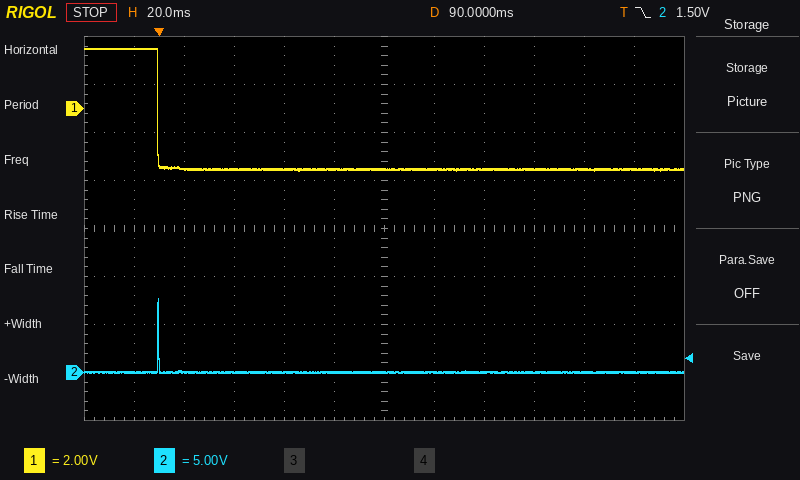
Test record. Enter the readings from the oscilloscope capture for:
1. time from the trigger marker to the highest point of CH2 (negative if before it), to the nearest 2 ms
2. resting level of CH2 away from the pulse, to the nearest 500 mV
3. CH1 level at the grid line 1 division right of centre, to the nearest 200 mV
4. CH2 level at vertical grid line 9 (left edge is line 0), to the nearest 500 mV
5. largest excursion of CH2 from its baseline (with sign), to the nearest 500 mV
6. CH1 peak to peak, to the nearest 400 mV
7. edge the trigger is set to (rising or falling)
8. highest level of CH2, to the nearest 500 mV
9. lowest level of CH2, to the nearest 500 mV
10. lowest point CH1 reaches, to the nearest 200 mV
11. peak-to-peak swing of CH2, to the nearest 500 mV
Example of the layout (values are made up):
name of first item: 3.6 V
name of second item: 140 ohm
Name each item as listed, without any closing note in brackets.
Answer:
time from the trigger marker to the highest point of CH2 (negative if before it), to the nearest 2 ms: 0 ms
resting level of CH2 away from the pulse, to the nearest 500 mV: 0.0 V
CH1 level at the grid line 1 division right of centre, to the nearest 200 mV: -2.6 V
CH2 level at vertical grid line 9 (left edge is line 0), to the nearest 500 mV: 0.0 V
largest excursion of CH2 from its baseline (with sign), to the nearest 500 mV: +7.5 V
CH1 peak to peak, to the nearest 400 mV: 5.2 V
edge the trigger is set to: falling
highest level of CH2, to the nearest 500 mV: 7.5 V
lowest level of CH2, to the nearest 500 mV: 0.0 V
lowest point CH1 reaches, to the nearest 200 mV: -2.6 V
peak-to-peak swing of CH2, to the nearest 500 mV: 7.5 V
